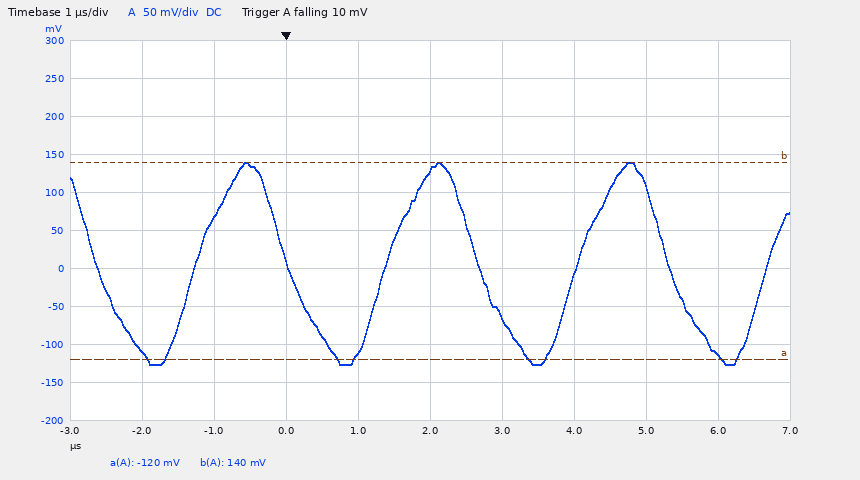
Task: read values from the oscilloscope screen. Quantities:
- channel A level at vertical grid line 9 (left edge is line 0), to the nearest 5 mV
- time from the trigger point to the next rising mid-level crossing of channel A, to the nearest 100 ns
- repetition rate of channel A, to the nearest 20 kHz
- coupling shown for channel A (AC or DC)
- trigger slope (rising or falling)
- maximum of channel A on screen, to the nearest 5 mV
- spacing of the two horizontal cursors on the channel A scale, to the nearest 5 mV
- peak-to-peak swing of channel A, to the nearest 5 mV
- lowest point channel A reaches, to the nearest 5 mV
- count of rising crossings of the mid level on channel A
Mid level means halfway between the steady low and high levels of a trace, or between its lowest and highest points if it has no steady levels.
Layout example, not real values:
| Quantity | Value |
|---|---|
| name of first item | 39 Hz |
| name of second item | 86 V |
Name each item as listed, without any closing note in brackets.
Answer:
| Quantity | Value |
|---|---|
| channel A level at vertical grid line 9 (left edge is line 0), to the nearest 5 mV | -115 mV |
| time from the trigger point to the next rising mid-level crossing of channel A, to the nearest 100 ns | 1.4 µs |
| repetition rate of channel A, to the nearest 20 kHz | 380 kHz |
| coupling shown for channel A | DC |
| trigger slope | falling |
| maximum of channel A on screen, to the nearest 5 mV | 140 mV |
| spacing of the two horizontal cursors on the channel A scale, to the nearest 5 mV | 260 mV |
| peak-to-peak swing of channel A, to the nearest 5 mV | 265 mV |
| lowest point channel A reaches, to the nearest 5 mV | -125 mV |
| count of rising crossings of the mid level on channel A | 4 |
